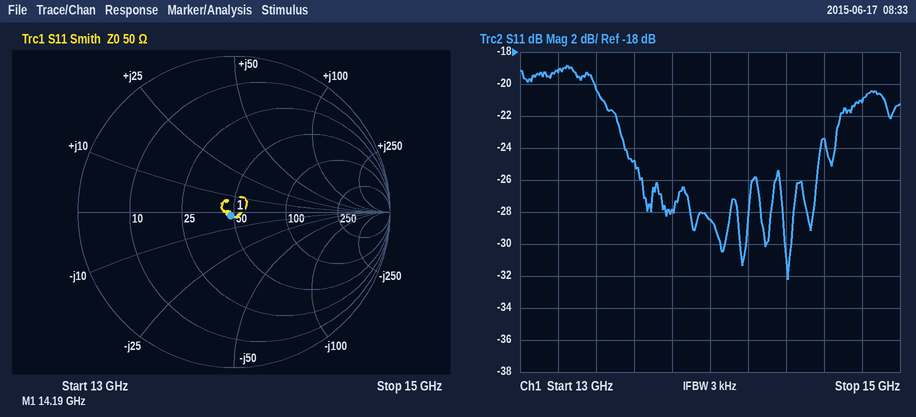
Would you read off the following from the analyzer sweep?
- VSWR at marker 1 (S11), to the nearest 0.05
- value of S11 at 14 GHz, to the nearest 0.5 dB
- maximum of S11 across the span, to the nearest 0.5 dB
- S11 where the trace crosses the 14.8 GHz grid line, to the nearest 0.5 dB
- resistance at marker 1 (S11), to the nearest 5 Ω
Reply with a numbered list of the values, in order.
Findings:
1. 1.05
2. -28.5 dB
3. -19.0 dB
4. -21.0 dB
5. 50 Ω
